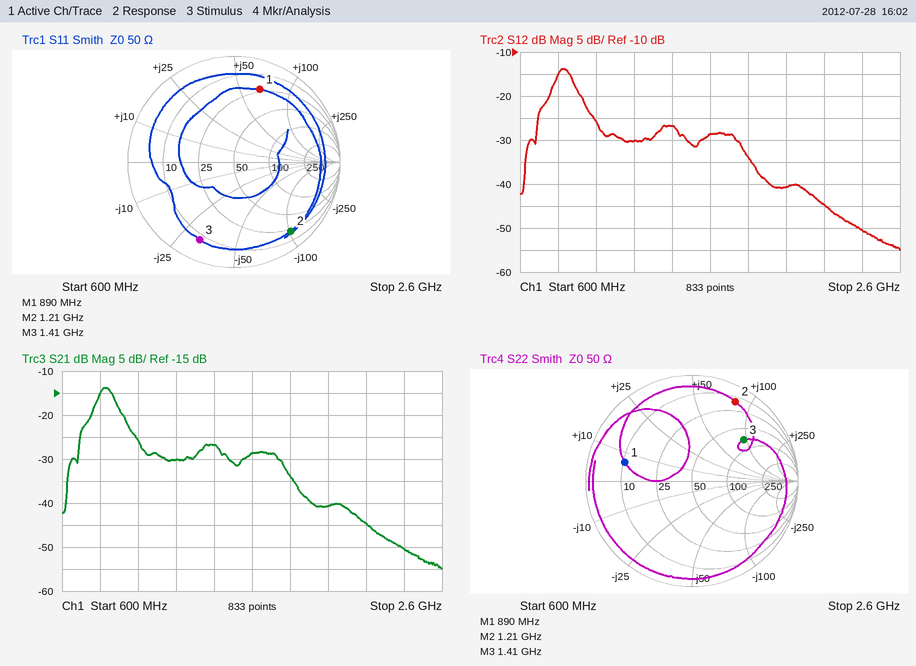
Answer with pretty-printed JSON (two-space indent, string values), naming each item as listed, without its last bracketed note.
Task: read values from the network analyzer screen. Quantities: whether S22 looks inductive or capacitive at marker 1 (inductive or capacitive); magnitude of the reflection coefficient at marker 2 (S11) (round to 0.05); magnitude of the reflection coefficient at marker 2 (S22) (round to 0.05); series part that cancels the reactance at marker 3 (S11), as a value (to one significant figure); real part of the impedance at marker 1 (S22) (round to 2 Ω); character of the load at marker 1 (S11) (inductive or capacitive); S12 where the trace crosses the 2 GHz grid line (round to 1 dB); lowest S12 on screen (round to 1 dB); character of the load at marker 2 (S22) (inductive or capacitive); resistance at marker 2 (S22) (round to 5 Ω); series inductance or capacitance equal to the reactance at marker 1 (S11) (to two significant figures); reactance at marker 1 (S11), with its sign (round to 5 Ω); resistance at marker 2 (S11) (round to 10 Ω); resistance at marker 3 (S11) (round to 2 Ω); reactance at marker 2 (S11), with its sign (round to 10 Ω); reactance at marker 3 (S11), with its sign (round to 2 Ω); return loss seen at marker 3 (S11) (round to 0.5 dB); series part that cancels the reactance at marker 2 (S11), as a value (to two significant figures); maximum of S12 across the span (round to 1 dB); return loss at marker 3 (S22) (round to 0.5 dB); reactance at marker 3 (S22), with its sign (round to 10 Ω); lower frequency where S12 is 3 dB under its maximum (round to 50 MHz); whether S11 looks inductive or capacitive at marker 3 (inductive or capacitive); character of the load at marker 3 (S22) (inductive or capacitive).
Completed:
{
  "whether S22 looks inductive or capacitive at marker 1": "inductive",
  "magnitude of the reflection coefficient at marker 2 (S11)": "0.85",
  "magnitude of the reflection coefficient at marker 2 (S22)": "0.85",
  "series part that cancels the reactance at marker 3 (S11), as a value": "4 nH",
  "real part of the impedance at marker 1 (S22)": "10 Ω",
  "character of the load at marker 1 (S11)": "inductive",
  "S12 where the trace crosses the 2 GHz grid line": "-41 dB",
  "lowest S12 on screen": "-55 dB",
  "character of the load at marker 2 (S22)": "inductive",
  "resistance at marker 2 (S22)": "15 Ω",
  "series inductance or capacitance equal to the reactance at marker 1 (S11)": "12 nH",
  "reactance at marker 1 (S11), with its sign": "+65 Ω",
  "resistance at marker 2 (S11)": "20 Ω",
  "resistance at marker 3 (S11)": "8 Ω",
  "reactance at marker 2 (S11), with its sign": "-100 Ω",
  "reactance at marker 3 (S11), with its sign": "-32 Ω",
  "return loss seen at marker 3 (S11)": "2.0 dB",
  "series part that cancels the reactance at marker 2 (S11), as a value": "13 nH",
  "maximum of S12 across the span": "-14 dB",
  "return loss at marker 3 (S22)": "4.0 dB",
  "reactance at marker 3 (S22), with its sign": "+90 Ω",
  "lower frequency where S12 is 3 dB under its maximum": "800 MHz",
  "whether S11 looks inductive or capacitive at marker 3": "capacitive",
  "character of the load at marker 3 (S22)": "inductive"
}
